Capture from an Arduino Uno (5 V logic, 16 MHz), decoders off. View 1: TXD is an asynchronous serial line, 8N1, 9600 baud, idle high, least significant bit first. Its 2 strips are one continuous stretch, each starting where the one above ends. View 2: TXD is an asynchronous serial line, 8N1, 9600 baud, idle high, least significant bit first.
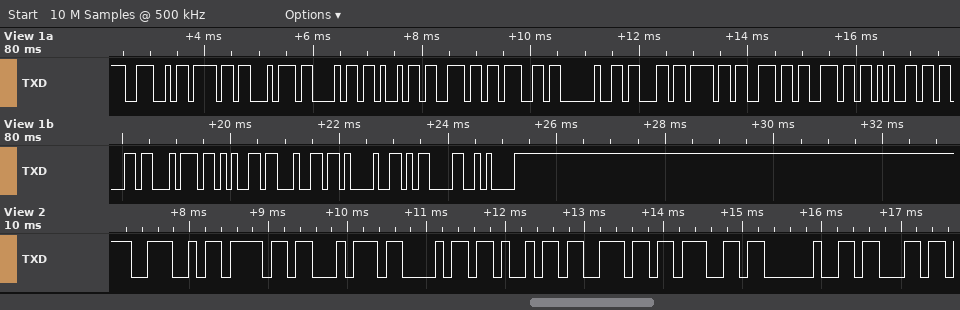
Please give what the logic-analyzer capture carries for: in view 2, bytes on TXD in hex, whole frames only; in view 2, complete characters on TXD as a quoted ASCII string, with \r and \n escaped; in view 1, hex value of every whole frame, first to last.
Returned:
0x4E 0x6F 0x74 0x68 0x69 0x6E 0x67 0x20 0x63
"Nothing c"
4E 6F 74 68 69 6E 67 20 63 6F 6E 6E 65 63 74 65 64 21 0D 0A
